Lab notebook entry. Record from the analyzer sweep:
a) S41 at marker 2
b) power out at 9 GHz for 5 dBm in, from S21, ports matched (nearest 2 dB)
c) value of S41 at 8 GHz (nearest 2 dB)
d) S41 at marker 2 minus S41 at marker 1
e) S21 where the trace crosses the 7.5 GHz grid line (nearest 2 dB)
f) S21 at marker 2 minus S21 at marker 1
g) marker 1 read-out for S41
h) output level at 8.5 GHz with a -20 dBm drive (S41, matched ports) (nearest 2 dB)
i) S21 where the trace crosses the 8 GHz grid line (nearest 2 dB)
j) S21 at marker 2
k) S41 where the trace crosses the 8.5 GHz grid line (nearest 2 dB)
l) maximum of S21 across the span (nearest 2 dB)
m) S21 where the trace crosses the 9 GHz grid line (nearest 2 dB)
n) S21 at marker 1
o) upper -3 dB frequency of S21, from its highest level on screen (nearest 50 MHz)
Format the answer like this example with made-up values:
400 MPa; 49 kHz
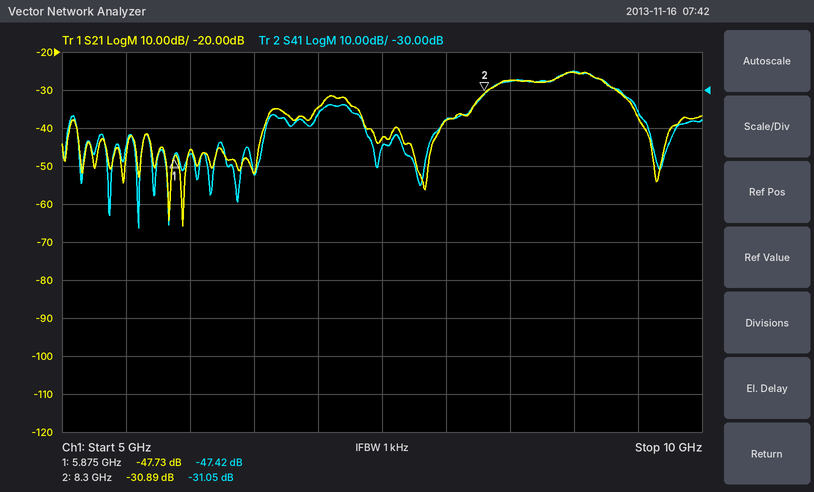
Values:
-31.05 dB; -20 dBm; -38 dB; 16.37 dB; -42 dB; 16.84 dB; -47.42 dB; -48 dBm; -38 dB; -30.89 dB; -28 dB; -26 dB; -26 dB; -47.73 dB; 9.25 GHz
